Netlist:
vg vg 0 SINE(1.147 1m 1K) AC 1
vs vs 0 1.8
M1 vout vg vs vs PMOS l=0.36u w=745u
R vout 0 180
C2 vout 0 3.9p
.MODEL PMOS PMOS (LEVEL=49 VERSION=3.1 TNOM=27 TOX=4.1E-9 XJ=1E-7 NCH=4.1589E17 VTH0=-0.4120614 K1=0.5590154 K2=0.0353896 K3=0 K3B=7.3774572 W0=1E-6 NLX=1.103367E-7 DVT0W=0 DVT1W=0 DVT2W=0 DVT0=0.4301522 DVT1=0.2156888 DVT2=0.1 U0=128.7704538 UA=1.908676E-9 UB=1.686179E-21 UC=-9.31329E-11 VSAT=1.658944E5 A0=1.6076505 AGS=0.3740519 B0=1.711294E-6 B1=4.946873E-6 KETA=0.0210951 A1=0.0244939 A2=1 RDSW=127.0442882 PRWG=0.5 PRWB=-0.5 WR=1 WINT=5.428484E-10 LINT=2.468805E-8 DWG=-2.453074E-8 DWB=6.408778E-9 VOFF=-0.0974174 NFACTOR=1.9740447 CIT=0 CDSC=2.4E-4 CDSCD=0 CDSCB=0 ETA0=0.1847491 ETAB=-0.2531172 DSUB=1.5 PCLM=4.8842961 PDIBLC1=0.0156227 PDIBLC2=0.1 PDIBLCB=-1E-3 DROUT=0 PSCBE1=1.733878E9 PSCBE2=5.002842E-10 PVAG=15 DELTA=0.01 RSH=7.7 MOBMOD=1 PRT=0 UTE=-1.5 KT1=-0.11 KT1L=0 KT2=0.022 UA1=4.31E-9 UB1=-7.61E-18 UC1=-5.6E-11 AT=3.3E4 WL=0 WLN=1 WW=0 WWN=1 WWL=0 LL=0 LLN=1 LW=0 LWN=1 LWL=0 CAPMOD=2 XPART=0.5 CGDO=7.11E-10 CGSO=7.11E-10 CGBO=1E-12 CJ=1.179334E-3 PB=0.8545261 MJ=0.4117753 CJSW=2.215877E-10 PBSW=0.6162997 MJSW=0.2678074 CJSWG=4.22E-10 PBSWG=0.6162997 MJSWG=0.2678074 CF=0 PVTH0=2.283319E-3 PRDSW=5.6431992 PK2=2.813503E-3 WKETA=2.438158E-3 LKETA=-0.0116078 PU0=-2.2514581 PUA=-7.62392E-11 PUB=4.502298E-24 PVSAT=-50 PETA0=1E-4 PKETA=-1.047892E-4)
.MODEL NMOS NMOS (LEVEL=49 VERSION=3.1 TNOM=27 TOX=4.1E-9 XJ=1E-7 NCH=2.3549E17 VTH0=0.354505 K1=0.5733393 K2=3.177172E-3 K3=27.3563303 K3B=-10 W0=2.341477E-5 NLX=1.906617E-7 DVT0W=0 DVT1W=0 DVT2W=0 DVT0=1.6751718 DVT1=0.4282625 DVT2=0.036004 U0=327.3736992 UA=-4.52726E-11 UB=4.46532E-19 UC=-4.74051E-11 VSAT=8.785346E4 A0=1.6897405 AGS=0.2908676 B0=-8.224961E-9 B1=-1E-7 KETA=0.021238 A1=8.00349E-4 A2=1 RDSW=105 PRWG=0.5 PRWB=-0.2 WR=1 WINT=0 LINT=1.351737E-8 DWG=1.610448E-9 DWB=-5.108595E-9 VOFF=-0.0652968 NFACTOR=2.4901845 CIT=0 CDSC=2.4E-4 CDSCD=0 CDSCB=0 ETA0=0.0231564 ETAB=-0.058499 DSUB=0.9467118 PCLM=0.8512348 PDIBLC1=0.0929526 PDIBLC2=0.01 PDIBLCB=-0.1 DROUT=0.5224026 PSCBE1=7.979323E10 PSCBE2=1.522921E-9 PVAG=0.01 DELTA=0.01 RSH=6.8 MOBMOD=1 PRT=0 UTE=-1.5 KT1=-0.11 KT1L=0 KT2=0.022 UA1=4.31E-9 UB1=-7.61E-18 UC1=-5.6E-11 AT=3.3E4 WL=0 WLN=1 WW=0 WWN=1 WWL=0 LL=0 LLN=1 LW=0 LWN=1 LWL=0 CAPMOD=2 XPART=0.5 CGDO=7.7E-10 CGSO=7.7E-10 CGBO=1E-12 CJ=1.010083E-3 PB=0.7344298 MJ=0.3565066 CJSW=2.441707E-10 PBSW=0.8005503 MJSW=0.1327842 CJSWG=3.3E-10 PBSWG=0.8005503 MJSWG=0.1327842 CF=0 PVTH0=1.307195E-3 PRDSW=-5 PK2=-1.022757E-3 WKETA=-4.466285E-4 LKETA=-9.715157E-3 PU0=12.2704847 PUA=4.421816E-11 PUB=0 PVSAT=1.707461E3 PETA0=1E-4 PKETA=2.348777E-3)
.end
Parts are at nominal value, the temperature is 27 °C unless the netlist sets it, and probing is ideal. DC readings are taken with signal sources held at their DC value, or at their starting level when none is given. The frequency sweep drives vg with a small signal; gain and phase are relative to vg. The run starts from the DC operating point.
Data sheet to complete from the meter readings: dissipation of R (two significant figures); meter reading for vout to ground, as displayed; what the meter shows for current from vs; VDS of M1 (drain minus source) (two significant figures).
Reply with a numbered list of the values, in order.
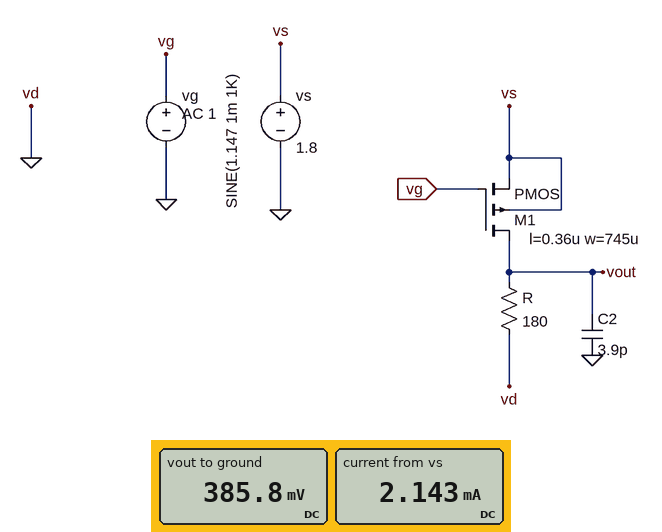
1. 830 µW
2. 385.8 mV
3. 2.143 mA
4. -1.4 V
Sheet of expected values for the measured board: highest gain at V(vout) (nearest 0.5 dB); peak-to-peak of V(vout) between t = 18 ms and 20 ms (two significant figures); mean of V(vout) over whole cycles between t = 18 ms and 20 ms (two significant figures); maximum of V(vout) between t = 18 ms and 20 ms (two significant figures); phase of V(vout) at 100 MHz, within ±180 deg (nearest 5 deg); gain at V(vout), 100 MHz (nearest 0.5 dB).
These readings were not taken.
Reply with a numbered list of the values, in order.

1. 10.5 dB
2. 6.8 mV
3. 390 mV
4. 390 mV
5. 150 deg
6. 9.5 dB
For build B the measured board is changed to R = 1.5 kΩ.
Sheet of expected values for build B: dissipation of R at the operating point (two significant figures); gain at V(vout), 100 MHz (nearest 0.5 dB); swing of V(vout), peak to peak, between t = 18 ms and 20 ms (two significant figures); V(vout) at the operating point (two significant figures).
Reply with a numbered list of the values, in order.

1. 2.0 mW
2. -6.0 dB
3. 1.0 mV
4. 1.7 V
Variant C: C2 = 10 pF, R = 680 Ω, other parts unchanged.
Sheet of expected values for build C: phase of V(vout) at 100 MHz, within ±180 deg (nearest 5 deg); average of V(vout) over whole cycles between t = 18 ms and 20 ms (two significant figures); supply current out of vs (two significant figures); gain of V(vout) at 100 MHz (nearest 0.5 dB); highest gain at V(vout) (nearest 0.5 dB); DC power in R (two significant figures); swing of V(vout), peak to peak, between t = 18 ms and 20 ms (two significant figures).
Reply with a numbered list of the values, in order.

1. 100 deg
2. 1.4 V
3. 2.0 mA
4. 8.5 dB
5. 21.0 dB
6. 2.7 mW
7. 22 mV
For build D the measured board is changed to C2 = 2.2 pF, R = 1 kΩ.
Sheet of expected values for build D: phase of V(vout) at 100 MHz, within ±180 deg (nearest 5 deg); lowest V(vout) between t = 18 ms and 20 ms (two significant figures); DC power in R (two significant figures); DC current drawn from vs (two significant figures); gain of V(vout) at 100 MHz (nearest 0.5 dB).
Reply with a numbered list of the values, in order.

1. 160 deg
2. 1.7 V
3. 2.8 mW
4. 1.7 mA
5. 4.0 dB
